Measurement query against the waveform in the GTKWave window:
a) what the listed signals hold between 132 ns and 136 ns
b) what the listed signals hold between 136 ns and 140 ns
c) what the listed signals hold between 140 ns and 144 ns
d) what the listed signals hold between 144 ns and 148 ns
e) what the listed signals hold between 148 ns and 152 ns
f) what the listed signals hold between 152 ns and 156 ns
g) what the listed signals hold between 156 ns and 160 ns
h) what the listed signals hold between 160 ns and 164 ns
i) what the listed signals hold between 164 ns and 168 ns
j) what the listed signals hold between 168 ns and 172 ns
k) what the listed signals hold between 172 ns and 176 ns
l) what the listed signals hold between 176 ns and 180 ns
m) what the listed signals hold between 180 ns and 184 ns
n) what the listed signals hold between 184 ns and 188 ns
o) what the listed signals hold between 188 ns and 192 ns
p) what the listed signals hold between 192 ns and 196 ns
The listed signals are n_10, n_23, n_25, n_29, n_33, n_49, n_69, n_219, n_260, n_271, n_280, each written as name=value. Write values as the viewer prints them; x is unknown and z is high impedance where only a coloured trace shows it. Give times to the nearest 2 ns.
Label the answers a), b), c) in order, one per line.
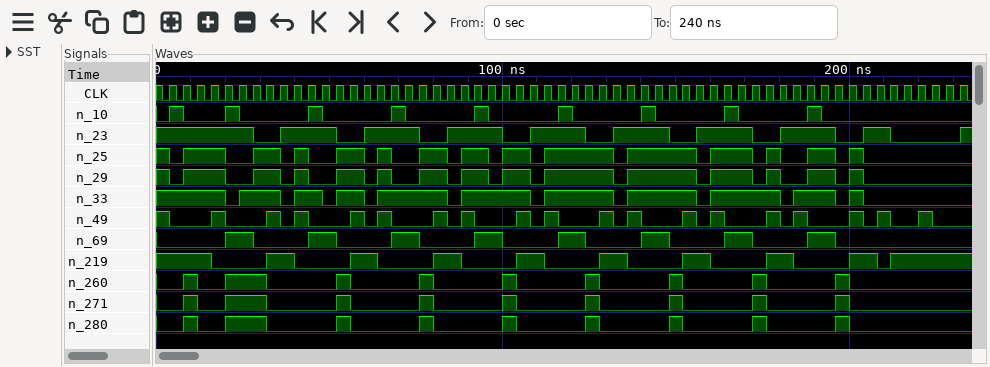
a) n_10=0, n_23=1, n_25=0, n_29=0, n_33=0, n_49=0, n_69=0, n_219=1, n_260=0, n_271=0, n_280=0
b) n_10=0, n_23=1, n_25=1, n_29=1, n_33=1, n_49=1, n_69=0, n_219=0, n_260=0, n_271=0, n_280=0
c) n_10=1, n_23=1, n_25=1, n_29=1, n_33=1, n_49=0, n_69=1, n_219=0, n_260=0, n_271=0, n_280=0
d) n_10=0, n_23=1, n_25=1, n_29=1, n_33=1, n_49=0, n_69=1, n_219=0, n_260=0, n_271=0, n_280=0
e) n_10=0, n_23=0, n_25=1, n_29=1, n_33=1, n_49=0, n_69=0, n_219=0, n_260=1, n_271=1, n_280=1
f) n_10=0, n_23=0, n_25=1, n_29=1, n_33=1, n_49=1, n_69=0, n_219=1, n_260=0, n_271=0, n_280=0
g) n_10=0, n_23=1, n_25=0, n_29=0, n_33=0, n_49=0, n_69=0, n_219=1, n_260=0, n_271=0, n_280=0
h) n_10=0, n_23=1, n_25=1, n_29=1, n_33=1, n_49=1, n_69=0, n_219=0, n_260=0, n_271=0, n_280=0
i) n_10=1, n_23=1, n_25=1, n_29=1, n_33=1, n_49=0, n_69=1, n_219=0, n_260=0, n_271=0, n_280=0
j) n_10=0, n_23=1, n_25=1, n_29=1, n_33=1, n_49=0, n_69=1, n_219=0, n_260=0, n_271=0, n_280=0
k) n_10=0, n_23=0, n_25=0, n_29=0, n_33=1, n_49=0, n_69=0, n_219=0, n_260=1, n_271=1, n_280=1
l) n_10=0, n_23=0, n_25=1, n_29=1, n_33=1, n_49=1, n_69=0, n_219=1, n_260=0, n_271=0, n_280=0
m) n_10=0, n_23=1, n_25=0, n_29=0, n_33=0, n_49=0, n_69=0, n_219=1, n_260=0, n_271=0, n_280=0
n) n_10=0, n_23=1, n_25=0, n_29=0, n_33=1, n_49=1, n_69=0, n_219=0, n_260=0, n_271=0, n_280=0
o) n_10=1, n_23=1, n_25=1, n_29=1, n_33=1, n_49=0, n_69=1, n_219=0, n_260=0, n_271=0, n_280=0
p) n_10=0, n_23=1, n_25=1, n_29=1, n_33=1, n_49=0, n_69=1, n_219=0, n_260=0, n_271=0, n_280=0
